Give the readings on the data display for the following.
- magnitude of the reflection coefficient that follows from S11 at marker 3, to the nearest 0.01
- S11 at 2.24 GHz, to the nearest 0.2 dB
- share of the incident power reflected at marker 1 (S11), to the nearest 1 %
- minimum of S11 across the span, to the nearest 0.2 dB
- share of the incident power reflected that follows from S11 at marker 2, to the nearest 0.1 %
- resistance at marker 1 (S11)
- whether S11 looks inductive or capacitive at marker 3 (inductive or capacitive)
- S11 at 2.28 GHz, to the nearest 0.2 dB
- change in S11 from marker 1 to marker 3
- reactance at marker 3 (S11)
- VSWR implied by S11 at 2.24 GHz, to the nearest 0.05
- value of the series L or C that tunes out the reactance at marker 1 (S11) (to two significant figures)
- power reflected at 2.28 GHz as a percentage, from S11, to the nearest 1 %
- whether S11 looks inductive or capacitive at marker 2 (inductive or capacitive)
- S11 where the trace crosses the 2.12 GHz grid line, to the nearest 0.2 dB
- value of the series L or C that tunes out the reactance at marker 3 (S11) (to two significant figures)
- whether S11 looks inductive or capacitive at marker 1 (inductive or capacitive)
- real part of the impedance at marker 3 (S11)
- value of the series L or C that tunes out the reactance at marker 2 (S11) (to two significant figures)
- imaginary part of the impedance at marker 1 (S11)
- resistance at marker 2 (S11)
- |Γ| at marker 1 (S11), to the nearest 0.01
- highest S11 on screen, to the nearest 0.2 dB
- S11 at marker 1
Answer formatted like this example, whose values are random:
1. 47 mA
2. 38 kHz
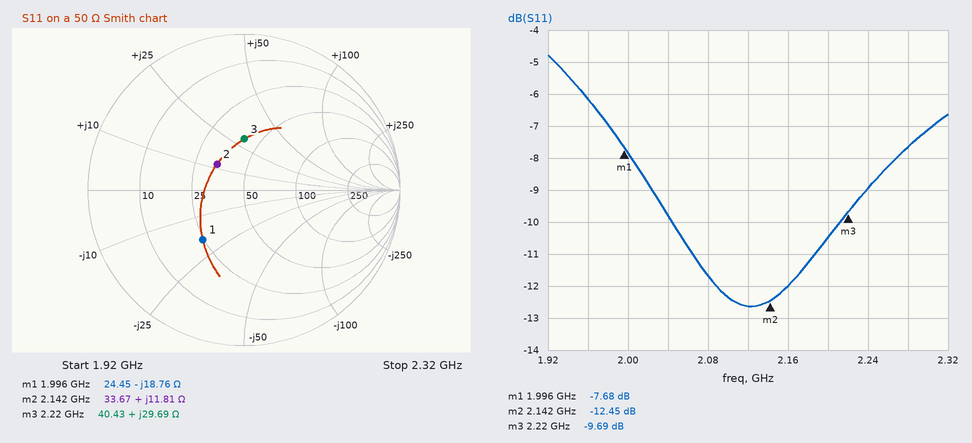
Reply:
1. 0.33
2. -9.0 dB
3. 17 %
4. -12.6 dB
5. 5.7 %
6. 24.45 Ω
7. inductive
8. -7.6 dB
9. -2.01 dB
10. +29.69 Ω
11. 2.10
12. 1.5 nH
13. 17 %
14. inductive
15. -12.6 dB
16. 2.4 pF
17. capacitive
18. 40.43 Ω
19. 6.3 pF
20. -18.76 Ω
21. 33.67 Ω
22. 0.41
23. -4.8 dB
24. -7.68 dB
